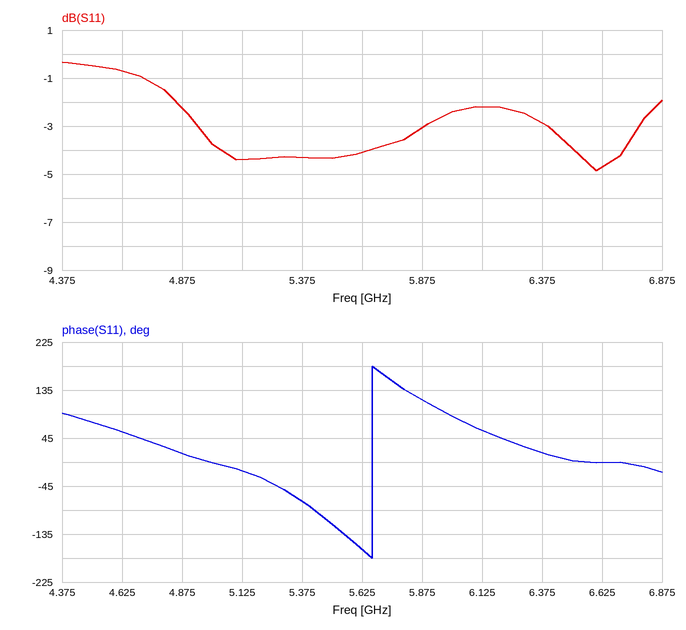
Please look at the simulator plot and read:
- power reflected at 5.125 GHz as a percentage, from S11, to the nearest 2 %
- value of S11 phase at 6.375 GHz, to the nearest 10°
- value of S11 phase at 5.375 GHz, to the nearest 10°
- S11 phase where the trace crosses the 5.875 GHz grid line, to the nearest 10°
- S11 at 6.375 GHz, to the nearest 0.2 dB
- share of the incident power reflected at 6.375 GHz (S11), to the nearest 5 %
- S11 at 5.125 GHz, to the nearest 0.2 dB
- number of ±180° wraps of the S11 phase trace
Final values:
36 %
20°
-70°
120°
-2.8 dB
50 %
-4.4 dB
1
